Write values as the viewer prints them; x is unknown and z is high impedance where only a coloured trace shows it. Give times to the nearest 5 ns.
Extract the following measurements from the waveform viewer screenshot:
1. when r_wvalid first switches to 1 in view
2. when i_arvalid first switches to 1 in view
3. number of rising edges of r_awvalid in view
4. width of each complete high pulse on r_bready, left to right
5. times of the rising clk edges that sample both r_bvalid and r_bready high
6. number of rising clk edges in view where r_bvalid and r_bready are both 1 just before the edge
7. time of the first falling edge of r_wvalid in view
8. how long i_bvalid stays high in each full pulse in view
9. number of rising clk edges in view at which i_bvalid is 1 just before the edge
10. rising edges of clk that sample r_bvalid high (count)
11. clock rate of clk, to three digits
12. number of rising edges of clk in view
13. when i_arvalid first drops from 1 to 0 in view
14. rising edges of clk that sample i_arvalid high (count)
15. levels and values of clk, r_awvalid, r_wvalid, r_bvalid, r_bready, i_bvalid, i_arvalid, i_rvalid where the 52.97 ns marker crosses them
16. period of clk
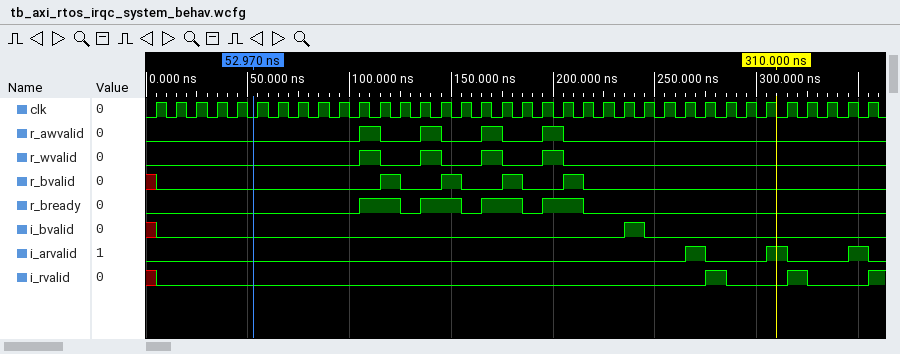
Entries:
105 ns
265 ns
4
20 ns, 20 ns, 20 ns, 20 ns
125 ns, 155 ns, 185 ns, 215 ns
4
115 ns
10 ns
1
4
100 MHz
36
275 ns
3
clk=0, r_awvalid=0, r_wvalid=0, r_bvalid=0, r_bready=0, i_bvalid=0, i_arvalid=0, i_rvalid=0
10 ns
